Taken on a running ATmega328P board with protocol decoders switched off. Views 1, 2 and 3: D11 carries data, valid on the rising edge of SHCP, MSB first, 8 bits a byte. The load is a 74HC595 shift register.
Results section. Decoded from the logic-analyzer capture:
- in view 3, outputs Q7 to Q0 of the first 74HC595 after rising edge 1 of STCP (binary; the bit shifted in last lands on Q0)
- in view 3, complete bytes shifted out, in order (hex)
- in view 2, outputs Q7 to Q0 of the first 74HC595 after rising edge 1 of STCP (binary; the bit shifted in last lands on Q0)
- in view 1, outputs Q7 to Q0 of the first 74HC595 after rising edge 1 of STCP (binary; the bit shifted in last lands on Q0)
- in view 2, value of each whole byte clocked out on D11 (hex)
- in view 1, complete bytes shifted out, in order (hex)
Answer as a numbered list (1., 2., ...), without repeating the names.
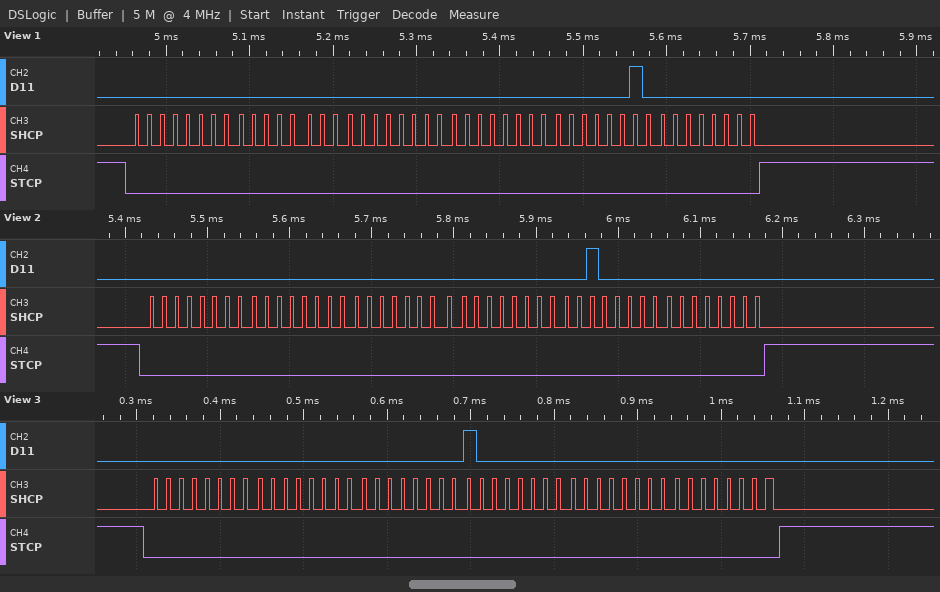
1. 00000000
2. 00 00 00 80 00 00
3. 00000000
4. 00000000
5. 00 00 00 00 20 00
6. 0x00 0x00 0x00 0x00 0x02 0x00
